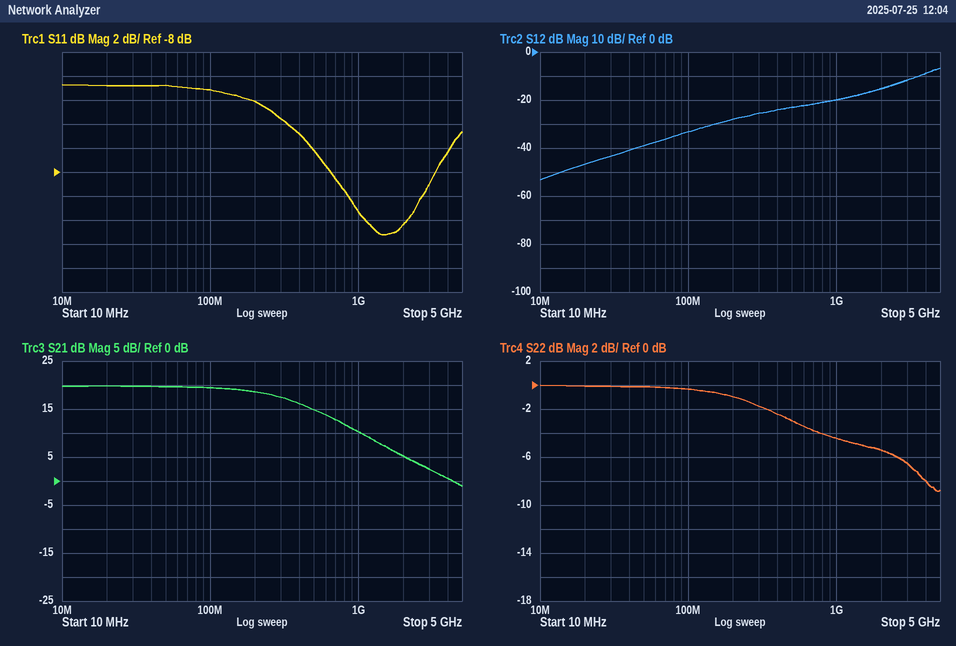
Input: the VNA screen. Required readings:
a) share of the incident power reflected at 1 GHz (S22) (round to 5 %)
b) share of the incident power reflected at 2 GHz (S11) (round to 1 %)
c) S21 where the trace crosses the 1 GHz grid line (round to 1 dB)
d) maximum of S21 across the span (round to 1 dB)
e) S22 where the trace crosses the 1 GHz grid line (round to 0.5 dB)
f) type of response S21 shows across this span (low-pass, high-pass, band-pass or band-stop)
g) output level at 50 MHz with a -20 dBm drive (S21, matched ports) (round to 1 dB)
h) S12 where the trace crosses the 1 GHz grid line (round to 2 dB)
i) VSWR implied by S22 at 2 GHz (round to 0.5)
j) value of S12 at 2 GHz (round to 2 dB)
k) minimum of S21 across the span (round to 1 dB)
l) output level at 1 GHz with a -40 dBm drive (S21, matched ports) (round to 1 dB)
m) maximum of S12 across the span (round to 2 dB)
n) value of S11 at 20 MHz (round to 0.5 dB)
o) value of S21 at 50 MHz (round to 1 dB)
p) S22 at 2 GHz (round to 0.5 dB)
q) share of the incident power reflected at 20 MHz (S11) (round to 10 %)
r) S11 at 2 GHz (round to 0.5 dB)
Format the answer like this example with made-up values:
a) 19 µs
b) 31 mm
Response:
a) 35 %
b) 6 %
c) 10 dB
d) 20 dB
e) -4.5 dB
f) low-pass
g) 0 dBm
h) -20 dB
i) 3.5
j) -16 dB
k) -1 dB
l) -30 dBm
m) -6 dB
n) -1.0 dB
o) 20 dB
p) -5.5 dB
q) 80 %
r) -12.5 dB
